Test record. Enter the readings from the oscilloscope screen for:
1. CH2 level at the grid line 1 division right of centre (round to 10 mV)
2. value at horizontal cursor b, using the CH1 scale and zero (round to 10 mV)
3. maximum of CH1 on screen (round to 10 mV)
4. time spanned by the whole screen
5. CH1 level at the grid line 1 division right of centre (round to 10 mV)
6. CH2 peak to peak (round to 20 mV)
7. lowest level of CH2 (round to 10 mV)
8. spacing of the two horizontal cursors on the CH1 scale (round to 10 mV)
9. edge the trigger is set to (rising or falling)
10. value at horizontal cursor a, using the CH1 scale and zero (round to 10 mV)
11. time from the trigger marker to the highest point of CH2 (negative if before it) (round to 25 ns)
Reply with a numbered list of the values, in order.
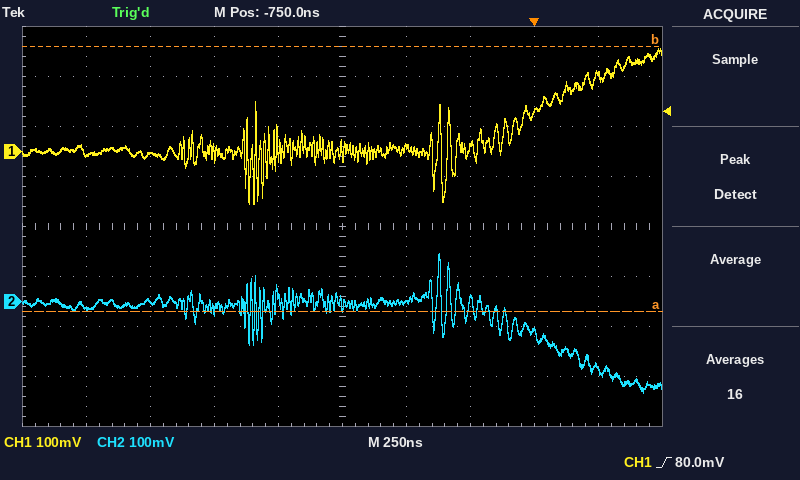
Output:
1. 0 mV
2. 210 mV
3. 210 mV
4. 2.5 µs
5. 10 mV
6. 280 mV
7. -180 mV
8. 530 mV
9. rising
10. -320 mV
11. -375 ns
